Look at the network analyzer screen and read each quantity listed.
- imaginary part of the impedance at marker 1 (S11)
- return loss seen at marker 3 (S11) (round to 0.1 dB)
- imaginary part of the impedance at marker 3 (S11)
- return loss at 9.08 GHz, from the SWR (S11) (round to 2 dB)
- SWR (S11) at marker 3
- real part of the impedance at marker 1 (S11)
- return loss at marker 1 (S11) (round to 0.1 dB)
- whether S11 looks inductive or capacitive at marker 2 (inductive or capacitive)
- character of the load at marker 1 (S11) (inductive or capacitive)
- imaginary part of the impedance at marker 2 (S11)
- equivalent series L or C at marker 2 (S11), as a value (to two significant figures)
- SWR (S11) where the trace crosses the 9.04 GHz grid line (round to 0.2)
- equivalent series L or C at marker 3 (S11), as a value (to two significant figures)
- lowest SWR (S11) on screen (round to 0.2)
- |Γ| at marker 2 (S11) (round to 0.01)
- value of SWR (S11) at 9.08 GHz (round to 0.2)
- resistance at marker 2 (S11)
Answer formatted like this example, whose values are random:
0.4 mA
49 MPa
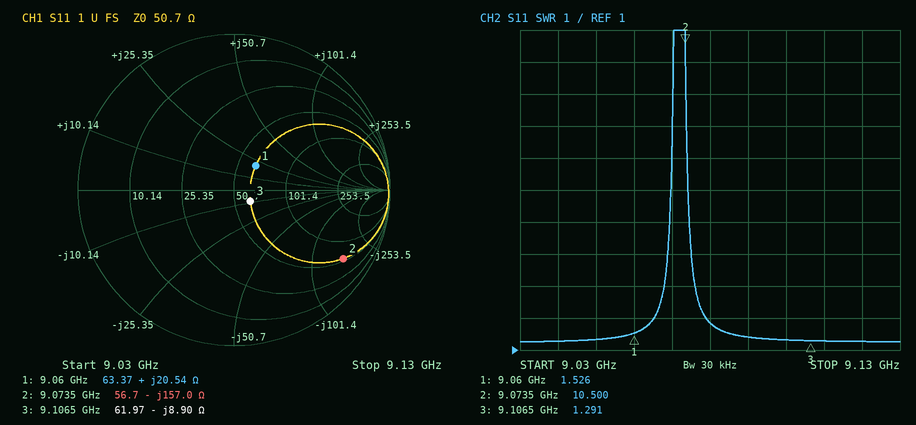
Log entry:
+20.54 Ω
17.9 dB
-8.90 Ω
10 dB
1.291
63.37 Ω
13.6 dB
capacitive
inductive
-157.0 Ω
110 fF
1.2
2.0 pF
1.2
0.83
1.8
56.7 Ω
